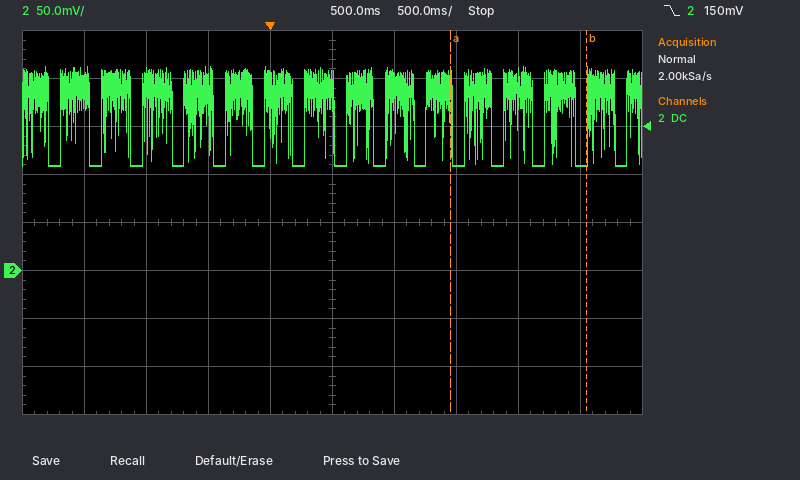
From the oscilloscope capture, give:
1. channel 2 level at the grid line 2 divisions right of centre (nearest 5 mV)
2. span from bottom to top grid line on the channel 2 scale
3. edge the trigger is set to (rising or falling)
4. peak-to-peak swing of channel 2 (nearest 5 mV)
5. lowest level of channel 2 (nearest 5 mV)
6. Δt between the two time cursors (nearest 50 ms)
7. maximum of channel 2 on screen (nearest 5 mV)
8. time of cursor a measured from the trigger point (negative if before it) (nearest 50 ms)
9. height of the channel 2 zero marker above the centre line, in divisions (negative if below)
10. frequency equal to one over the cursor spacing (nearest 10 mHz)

110 mV
400 mV
falling
105 mV
110 mV
1.10 s
215 mV
+1.45 s
-1.0 div
910 mHz
